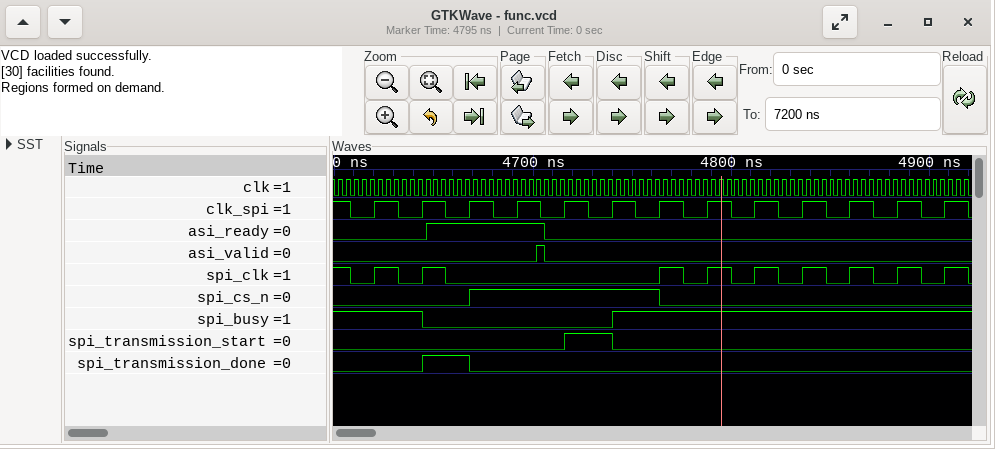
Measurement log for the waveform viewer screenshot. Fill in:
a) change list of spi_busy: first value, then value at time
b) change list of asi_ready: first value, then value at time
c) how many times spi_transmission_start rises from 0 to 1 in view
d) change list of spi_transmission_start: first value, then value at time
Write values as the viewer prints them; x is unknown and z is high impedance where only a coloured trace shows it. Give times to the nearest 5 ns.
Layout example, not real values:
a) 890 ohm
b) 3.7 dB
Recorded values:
a) 1, 0 at 4645 ns, 1 at 4740 ns
b) 0, 1 at 4645 ns, 0 at 4705 ns
c) 1
d) 0, 1 at 4715 ns, 0 at 4740 ns
